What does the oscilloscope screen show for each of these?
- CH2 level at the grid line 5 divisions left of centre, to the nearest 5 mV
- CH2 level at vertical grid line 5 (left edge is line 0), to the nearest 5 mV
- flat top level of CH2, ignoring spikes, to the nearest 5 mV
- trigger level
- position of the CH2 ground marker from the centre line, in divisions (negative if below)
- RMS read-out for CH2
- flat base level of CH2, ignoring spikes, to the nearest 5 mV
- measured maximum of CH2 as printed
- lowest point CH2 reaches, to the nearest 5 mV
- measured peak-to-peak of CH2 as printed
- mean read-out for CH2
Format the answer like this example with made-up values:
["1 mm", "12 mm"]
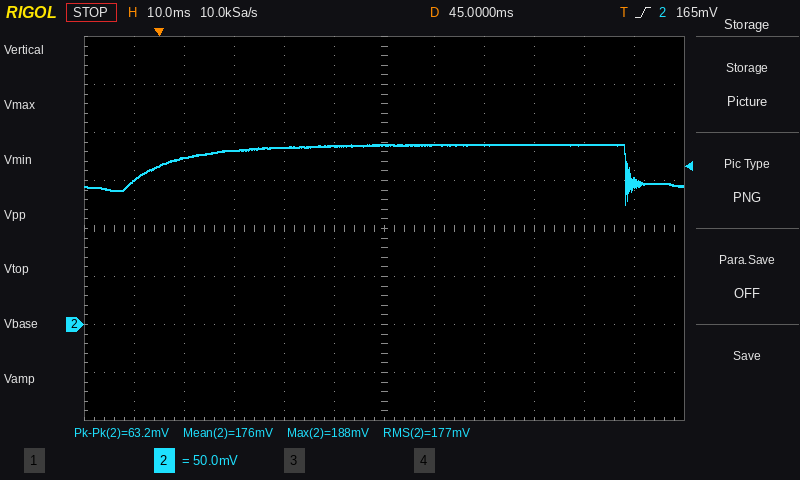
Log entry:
["150 mV", "185 mV", "185 mV", "165 mV", "-2.0 div", "177 mV", "145 mV", "188 mV", "125 mV", "63.2 mV", "176 mV"]
